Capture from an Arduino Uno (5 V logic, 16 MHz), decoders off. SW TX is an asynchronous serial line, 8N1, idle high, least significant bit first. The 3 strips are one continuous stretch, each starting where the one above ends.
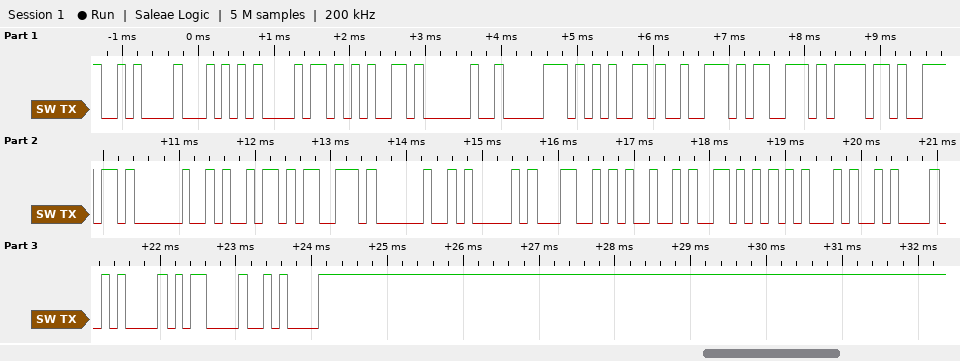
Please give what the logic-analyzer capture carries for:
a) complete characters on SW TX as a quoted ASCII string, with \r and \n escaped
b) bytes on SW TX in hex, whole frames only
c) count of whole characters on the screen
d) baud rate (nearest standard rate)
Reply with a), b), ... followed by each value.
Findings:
a) "\nThe person is ALIVE\n\n\r\n"
b) 0A 54 68 65 20 70 65 72 73 6F 6E 20 69 73 20 41 4C 49 56 45 0A 0A 0D 0A
c) 24
d) 9600 baud
